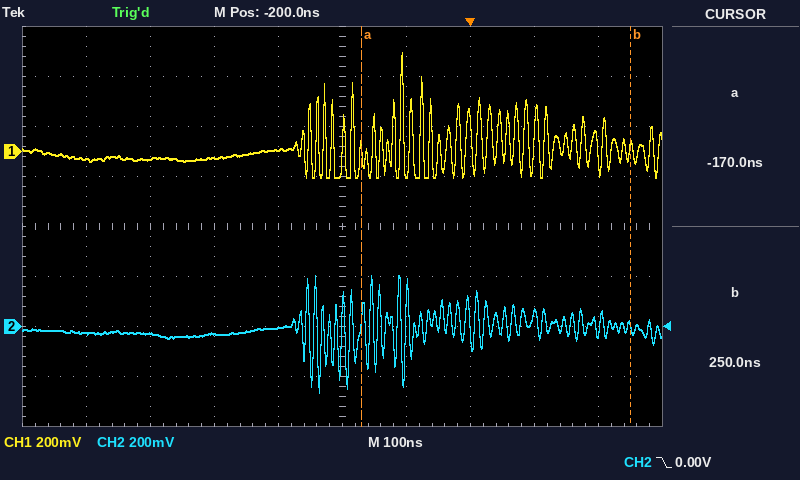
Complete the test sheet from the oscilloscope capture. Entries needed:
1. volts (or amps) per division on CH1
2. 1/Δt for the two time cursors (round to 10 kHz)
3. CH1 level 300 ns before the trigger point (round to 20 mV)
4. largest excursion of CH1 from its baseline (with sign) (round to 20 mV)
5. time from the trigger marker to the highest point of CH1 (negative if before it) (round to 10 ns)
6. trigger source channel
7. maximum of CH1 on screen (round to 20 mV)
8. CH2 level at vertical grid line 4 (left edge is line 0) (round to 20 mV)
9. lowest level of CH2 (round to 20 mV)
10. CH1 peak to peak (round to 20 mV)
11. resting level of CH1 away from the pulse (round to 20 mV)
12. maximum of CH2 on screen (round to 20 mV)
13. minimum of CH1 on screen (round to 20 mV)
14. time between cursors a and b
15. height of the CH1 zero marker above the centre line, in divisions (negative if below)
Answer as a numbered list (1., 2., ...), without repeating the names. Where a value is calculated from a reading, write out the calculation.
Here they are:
1. 200 mV
2. 1 / 420 ns ≈ 2.38 MHz
3. 0 mV
4. 400 mV − (-20 mV) = +420 mV
5. -110 ns
6. CH2
7. 400 mV
8. 0 mV
9. -260 mV
10. 400 mV − (-100 mV) = 500 mV
11. -20 mV
12. 200 mV
13. -100 mV
14. 250 ns − (-170 ns) = 420 ns
15. +1.5 div
